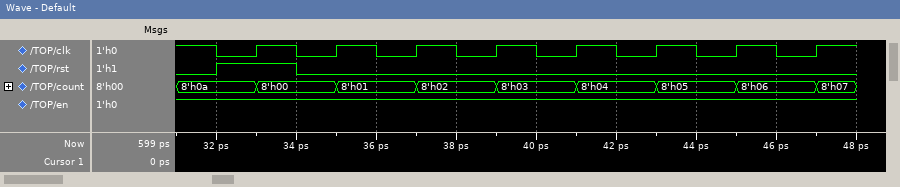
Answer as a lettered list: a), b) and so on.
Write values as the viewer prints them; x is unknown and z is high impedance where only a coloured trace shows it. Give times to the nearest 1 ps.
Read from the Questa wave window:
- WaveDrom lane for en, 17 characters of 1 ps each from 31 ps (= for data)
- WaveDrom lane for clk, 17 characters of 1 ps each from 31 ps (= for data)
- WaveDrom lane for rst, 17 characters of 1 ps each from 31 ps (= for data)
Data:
a) {name: 'en', wave: '1................'}
b) {name: 'clk', wave: '10101010101010101'}
c) {name: 'rst', wave: '01.0.............'}
